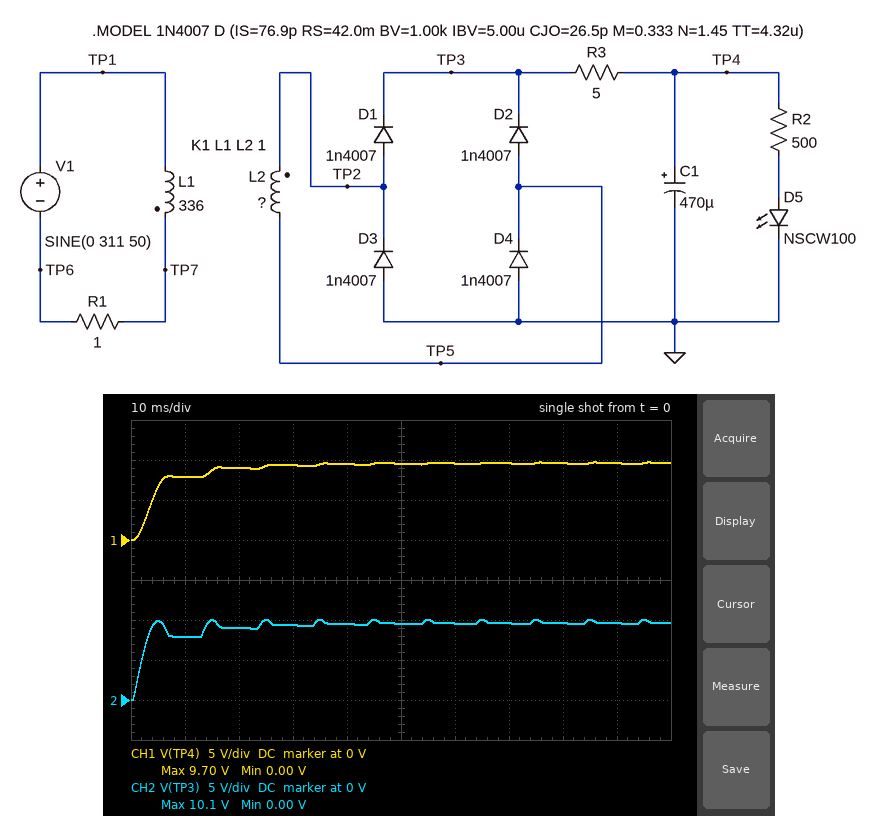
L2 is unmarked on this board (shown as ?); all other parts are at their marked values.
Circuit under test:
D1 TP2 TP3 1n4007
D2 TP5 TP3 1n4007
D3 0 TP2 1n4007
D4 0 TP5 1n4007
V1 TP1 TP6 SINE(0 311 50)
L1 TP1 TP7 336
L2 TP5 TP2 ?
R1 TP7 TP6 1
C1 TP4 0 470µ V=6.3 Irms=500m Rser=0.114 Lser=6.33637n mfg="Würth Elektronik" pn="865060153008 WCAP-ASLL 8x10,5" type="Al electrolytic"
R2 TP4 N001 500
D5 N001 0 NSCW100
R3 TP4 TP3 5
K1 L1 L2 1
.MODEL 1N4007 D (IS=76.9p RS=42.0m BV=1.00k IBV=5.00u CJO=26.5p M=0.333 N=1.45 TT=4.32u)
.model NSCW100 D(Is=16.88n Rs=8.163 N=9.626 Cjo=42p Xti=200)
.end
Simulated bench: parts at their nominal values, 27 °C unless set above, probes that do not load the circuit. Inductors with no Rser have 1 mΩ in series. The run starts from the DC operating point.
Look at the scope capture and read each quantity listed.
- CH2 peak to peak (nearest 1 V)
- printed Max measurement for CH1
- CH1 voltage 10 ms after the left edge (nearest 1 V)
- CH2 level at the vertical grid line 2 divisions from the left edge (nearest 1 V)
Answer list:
10 V
9.70 V
8 V
9 V
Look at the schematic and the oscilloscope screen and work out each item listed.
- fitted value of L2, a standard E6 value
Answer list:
470 mH
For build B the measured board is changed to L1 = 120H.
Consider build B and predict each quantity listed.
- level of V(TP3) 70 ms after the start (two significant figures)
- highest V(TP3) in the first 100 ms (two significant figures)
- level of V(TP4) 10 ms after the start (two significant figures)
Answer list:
17 V
18 V
14 V
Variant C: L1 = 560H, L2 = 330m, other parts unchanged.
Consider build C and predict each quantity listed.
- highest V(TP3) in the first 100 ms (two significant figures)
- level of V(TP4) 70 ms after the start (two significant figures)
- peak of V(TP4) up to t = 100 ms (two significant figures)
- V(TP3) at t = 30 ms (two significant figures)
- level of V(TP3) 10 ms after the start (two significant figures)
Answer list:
6.0 V
5.8 V
5.9 V
5.6 V
4.6 V
